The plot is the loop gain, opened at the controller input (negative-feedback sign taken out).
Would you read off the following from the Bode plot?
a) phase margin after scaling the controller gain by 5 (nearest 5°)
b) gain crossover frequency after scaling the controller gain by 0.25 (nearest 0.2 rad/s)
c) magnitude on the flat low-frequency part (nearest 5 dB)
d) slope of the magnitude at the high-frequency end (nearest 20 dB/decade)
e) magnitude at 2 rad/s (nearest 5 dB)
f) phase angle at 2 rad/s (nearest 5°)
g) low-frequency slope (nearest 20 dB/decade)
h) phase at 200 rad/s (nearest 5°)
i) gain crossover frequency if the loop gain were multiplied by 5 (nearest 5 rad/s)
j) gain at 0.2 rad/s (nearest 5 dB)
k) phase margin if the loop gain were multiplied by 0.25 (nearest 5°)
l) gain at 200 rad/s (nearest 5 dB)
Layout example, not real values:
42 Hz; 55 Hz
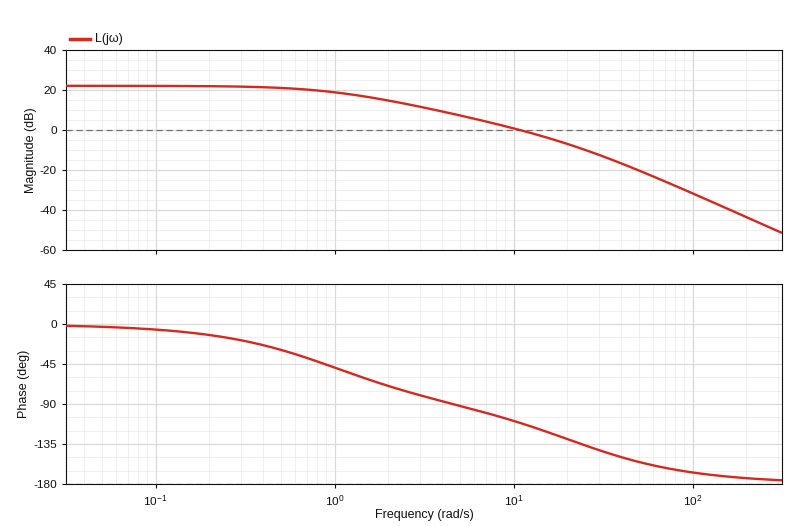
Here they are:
35°; 2.8 rad/s; 20 dB; -40 dB/decade; 15 dB; -70°; 0 dB/decade; -175°; 35 rad/s; 20 dB; 100°; -45 dB
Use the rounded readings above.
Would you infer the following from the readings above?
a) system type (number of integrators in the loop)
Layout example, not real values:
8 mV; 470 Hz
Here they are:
0
